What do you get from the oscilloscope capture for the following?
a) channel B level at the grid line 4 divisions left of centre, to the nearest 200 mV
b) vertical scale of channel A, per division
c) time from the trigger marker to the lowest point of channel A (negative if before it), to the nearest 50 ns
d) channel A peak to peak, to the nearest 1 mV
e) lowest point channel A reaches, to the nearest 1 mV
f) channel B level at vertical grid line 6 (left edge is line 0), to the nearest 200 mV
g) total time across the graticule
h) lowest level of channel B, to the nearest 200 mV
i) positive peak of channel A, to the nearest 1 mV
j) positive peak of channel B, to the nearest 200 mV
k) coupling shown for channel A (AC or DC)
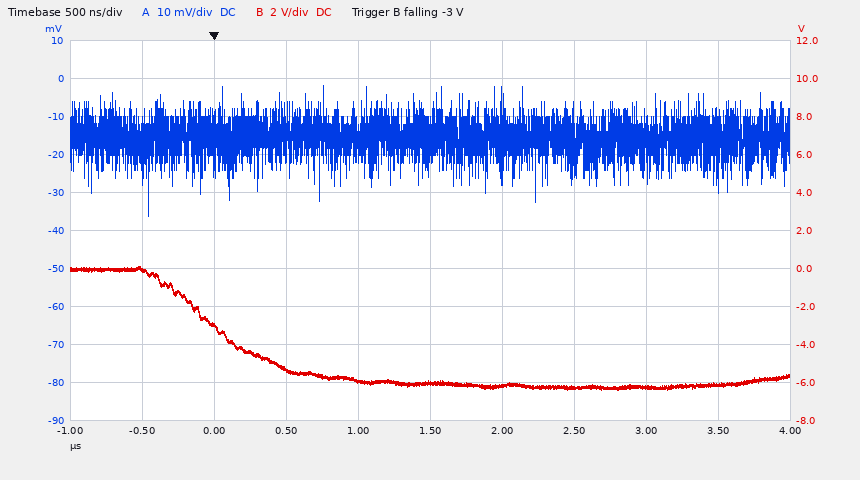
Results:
0.0 V
10 mV
-450 ns
34 mV
-36 mV
-6.2 V
5 µs
-6.4 V
-2 mV
200 mV
DC
